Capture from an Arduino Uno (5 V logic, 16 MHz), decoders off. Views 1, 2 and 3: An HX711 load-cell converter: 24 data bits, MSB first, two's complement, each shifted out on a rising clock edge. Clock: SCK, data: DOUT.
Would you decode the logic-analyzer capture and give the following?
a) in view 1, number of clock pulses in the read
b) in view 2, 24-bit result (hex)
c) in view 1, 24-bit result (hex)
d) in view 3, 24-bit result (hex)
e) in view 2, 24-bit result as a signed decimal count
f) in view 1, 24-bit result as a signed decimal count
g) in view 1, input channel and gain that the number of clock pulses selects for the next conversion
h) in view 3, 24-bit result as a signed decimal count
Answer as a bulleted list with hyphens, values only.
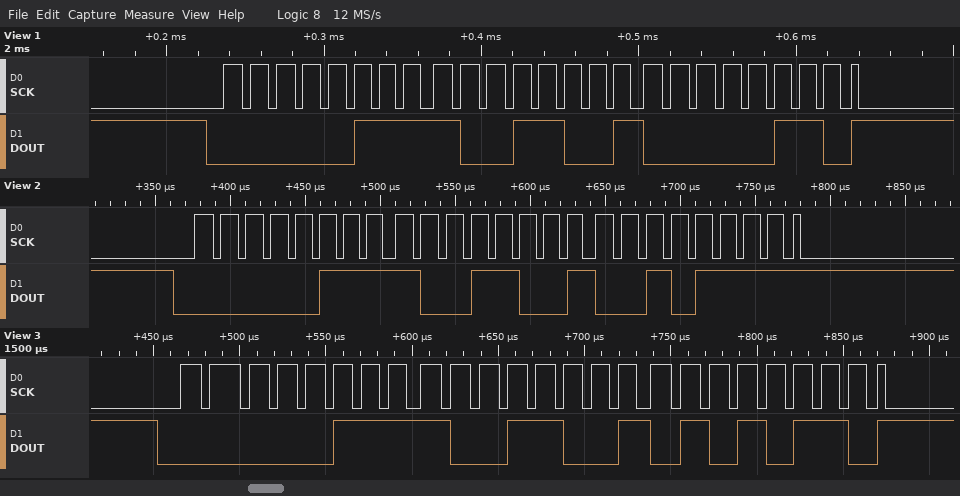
- 25
- 0x07992F
- 0x079906
- 0x079956
- 497967
- 497926
- channel A, gain 128
- 498006
